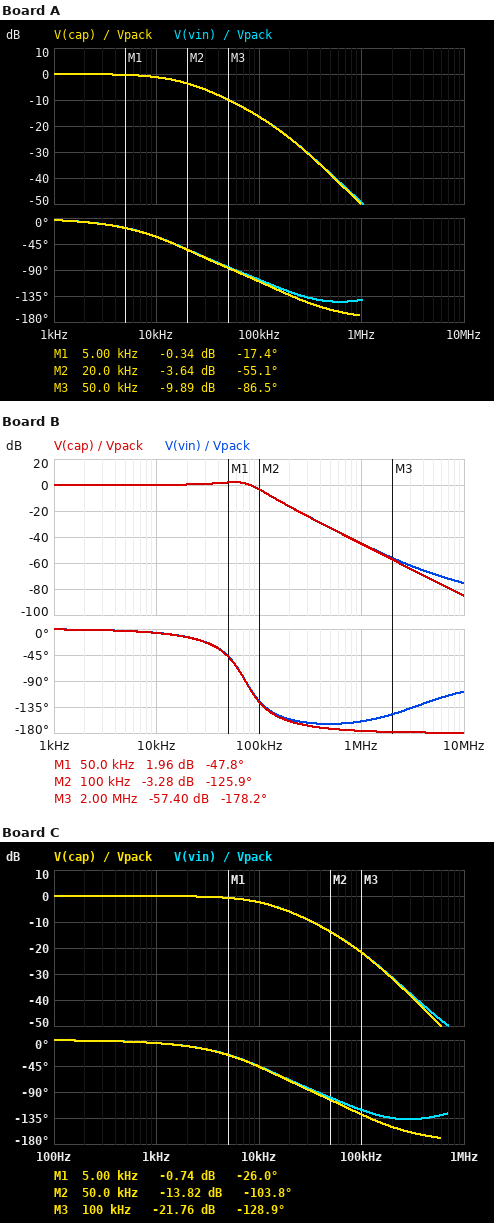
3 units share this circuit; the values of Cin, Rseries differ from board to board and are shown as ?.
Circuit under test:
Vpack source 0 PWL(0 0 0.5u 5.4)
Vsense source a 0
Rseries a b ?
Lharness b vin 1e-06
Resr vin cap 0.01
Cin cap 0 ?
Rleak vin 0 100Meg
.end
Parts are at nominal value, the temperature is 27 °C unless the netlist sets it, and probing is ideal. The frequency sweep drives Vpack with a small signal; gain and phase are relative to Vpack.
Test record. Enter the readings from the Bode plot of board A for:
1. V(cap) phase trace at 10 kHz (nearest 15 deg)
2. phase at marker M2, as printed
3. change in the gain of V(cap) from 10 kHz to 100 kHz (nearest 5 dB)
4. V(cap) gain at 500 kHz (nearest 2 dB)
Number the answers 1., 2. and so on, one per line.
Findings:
1. -30 deg
2. -55.1 deg
3. -15 dB
4. -38 dB
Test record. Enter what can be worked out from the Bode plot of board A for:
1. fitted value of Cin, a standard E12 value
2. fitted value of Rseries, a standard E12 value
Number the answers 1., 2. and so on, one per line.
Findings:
1. 8.2 µF
2. 1.2 Ω
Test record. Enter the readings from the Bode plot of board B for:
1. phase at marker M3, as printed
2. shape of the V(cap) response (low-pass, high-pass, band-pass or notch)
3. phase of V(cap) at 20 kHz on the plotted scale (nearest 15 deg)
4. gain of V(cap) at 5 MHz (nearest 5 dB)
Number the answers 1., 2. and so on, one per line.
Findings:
1. -178.2 deg
2. low-pass
3. -15 deg
4. -75 dB
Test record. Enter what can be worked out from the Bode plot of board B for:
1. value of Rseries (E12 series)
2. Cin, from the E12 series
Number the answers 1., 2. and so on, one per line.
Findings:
1. 0.39 Ω
2. 4.7 µF
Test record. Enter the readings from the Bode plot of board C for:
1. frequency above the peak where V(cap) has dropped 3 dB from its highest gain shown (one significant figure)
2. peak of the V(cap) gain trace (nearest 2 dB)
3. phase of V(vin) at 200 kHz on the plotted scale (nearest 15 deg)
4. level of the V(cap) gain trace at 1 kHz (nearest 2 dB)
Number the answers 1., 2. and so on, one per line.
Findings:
1. 10 kHz
2. 0 dB
3. -135 deg
4. 0 dB
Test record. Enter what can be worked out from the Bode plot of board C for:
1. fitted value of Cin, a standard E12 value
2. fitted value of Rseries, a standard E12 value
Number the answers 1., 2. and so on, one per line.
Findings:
1. 22 µF
2. 0.68 Ω
